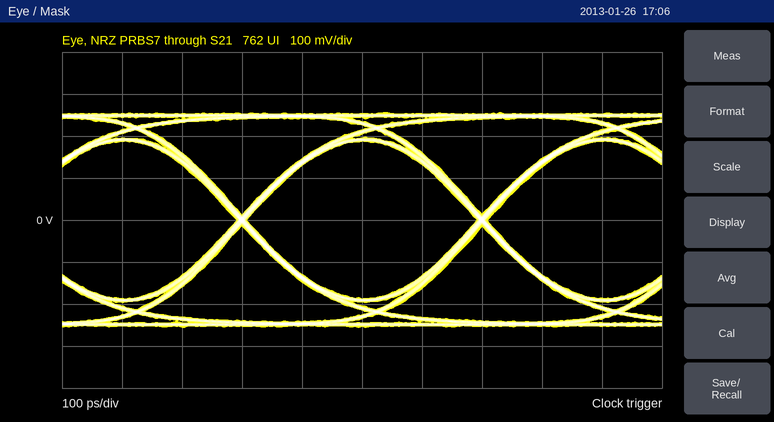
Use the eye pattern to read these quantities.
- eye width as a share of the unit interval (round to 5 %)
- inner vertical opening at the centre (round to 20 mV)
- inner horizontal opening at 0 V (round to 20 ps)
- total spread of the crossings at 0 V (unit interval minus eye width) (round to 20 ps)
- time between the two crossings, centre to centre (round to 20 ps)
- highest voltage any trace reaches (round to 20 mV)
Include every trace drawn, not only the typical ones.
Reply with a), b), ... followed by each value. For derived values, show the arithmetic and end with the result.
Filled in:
a) 380 ps / 400 ps ≈ 95 %
b) 380 mV
c) 380 ps
d) 20 ps
e) 400 ps
f) 260 mV
